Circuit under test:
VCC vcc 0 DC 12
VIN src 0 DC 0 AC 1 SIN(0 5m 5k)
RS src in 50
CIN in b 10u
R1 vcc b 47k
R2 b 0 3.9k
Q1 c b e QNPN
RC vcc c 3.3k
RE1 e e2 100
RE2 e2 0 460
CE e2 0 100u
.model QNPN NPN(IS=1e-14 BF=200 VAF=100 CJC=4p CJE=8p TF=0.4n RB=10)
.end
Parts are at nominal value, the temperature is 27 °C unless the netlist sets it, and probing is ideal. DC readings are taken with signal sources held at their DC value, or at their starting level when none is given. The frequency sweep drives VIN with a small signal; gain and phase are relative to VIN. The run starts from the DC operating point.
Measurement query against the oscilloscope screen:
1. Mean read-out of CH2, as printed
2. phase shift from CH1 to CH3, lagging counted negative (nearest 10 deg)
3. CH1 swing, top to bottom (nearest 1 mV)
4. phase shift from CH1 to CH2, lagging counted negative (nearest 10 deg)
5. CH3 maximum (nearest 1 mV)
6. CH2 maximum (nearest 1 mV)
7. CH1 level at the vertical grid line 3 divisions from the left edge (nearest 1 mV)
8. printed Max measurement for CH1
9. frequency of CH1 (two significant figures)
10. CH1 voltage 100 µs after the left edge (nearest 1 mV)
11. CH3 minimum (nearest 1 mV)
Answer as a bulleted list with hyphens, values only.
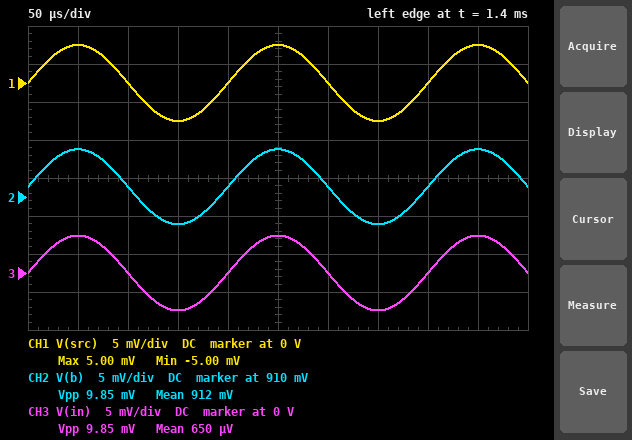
- 912 mV
- 0 deg
- 10 mV
- 0 deg
- 5 mV
- 916 mV
- -5 mV
- 5.00 mV
- 5.0 kHz
- 0 V
- -5 mV
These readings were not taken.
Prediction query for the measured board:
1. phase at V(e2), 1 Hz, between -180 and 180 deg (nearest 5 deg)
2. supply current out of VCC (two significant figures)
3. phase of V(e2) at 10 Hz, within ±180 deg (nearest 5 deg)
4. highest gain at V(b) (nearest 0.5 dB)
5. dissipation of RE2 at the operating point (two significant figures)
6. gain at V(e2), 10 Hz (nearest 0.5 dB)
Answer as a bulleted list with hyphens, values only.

- 75 deg
- 730 µA
- -10 deg
- 0 dB
- 110 µW
- -5.5 dB
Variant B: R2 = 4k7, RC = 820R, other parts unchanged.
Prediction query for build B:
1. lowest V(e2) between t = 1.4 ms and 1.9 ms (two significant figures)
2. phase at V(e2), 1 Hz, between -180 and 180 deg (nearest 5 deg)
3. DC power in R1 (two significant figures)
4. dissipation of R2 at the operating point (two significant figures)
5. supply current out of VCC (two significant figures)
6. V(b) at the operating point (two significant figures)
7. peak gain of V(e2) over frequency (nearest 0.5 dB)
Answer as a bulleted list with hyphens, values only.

- 350 mV
- 70 deg
- 2.5 mW
- 250 µW
- 1.0 mA
- 1.1 V
- -4.5 dB
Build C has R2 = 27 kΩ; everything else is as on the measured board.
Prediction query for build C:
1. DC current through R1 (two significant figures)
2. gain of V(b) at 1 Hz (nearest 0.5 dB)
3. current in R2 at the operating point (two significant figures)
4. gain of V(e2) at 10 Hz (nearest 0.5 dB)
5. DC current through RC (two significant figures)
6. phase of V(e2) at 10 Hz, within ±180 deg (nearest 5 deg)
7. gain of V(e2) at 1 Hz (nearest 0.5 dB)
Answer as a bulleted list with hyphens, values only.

- 200 µA
- -30.0 dB
- 91 µA
- -21.0 dB
- 3.1 mA
- 15 deg
- -32.0 dB
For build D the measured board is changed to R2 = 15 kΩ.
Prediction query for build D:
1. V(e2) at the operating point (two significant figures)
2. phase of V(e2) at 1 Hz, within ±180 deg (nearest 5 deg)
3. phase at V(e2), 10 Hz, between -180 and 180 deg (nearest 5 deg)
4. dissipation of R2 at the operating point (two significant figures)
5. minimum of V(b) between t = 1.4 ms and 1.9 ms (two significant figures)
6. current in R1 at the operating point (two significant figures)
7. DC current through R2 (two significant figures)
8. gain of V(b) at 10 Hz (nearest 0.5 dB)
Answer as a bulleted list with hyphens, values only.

- 1.4 V
- 75 deg
- 15 deg
- 390 µW
- 2.4 V
- 200 µA
- 160 µA
- -16.5 dB
